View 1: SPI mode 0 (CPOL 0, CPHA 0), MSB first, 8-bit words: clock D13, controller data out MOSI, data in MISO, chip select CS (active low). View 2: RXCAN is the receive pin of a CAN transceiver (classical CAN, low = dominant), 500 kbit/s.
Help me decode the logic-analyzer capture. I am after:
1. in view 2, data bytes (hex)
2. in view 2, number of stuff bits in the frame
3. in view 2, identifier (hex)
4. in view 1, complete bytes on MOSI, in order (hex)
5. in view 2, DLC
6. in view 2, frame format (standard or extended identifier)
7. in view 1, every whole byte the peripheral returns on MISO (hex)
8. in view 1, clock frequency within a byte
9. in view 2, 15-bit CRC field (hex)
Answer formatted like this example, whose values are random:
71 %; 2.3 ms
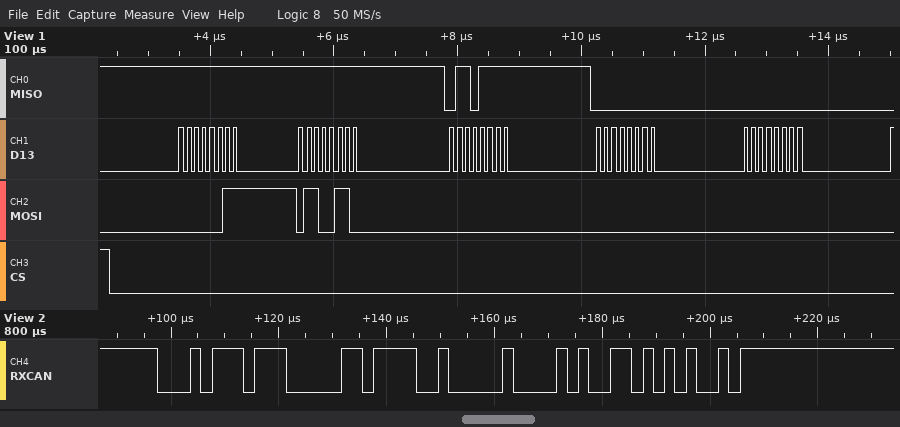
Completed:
F2 00; 2; 0x177; 03 66 00 00 00; 2; standard; FF FF 6F 00 00; 8 MHz; 0x5354
